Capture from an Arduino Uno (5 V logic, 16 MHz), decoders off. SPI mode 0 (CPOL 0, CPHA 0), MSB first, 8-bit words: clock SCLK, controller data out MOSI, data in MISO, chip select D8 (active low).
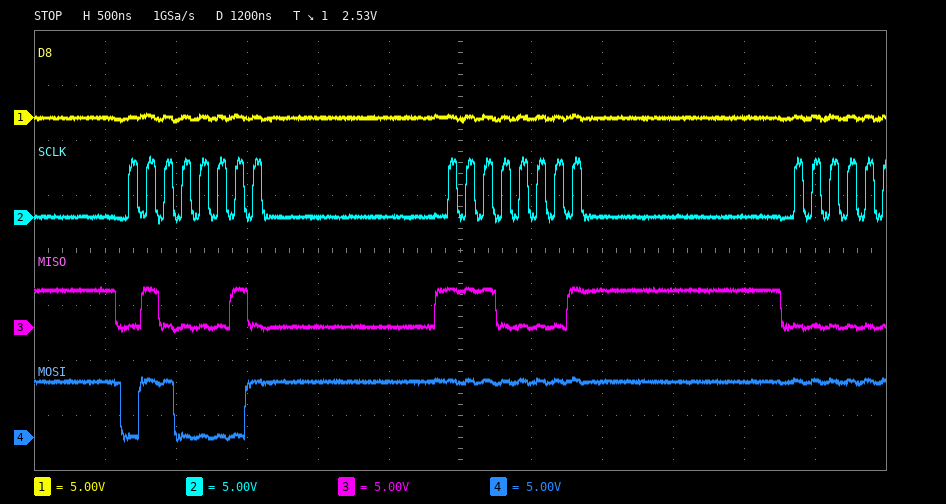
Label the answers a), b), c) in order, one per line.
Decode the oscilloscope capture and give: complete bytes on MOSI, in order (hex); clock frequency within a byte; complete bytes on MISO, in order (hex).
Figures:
a) 61 FF
b) 8 MHz
c) 42 E1
